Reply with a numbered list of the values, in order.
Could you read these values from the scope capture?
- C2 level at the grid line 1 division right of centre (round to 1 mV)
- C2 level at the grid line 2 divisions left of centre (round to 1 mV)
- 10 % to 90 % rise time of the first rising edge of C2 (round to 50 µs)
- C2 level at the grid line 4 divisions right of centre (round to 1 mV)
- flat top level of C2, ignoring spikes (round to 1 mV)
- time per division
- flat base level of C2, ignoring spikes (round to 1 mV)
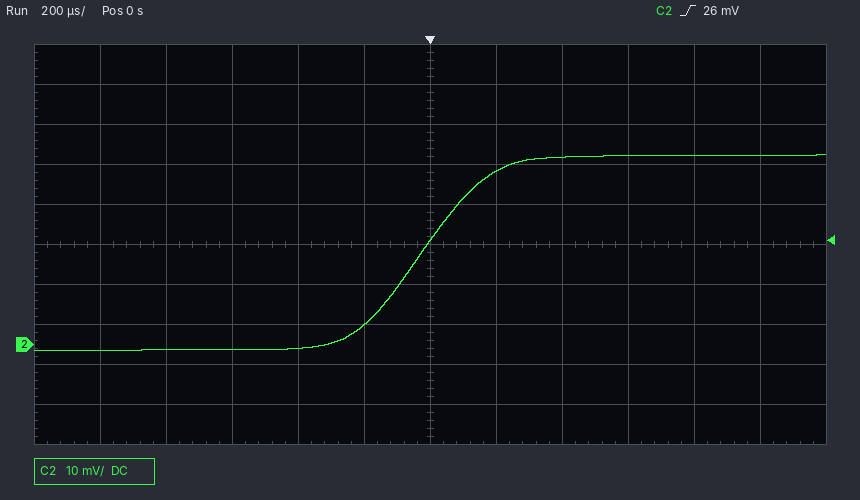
1. 43 mV
2. -1 mV
3. 400 µs
4. 47 mV
5. 47 mV
6. 200 µs
7. -1 mV
